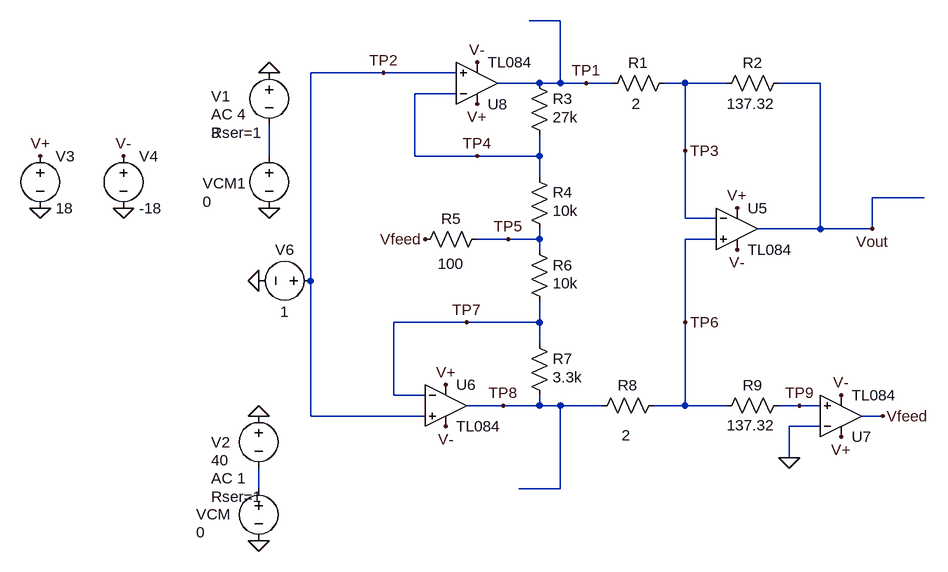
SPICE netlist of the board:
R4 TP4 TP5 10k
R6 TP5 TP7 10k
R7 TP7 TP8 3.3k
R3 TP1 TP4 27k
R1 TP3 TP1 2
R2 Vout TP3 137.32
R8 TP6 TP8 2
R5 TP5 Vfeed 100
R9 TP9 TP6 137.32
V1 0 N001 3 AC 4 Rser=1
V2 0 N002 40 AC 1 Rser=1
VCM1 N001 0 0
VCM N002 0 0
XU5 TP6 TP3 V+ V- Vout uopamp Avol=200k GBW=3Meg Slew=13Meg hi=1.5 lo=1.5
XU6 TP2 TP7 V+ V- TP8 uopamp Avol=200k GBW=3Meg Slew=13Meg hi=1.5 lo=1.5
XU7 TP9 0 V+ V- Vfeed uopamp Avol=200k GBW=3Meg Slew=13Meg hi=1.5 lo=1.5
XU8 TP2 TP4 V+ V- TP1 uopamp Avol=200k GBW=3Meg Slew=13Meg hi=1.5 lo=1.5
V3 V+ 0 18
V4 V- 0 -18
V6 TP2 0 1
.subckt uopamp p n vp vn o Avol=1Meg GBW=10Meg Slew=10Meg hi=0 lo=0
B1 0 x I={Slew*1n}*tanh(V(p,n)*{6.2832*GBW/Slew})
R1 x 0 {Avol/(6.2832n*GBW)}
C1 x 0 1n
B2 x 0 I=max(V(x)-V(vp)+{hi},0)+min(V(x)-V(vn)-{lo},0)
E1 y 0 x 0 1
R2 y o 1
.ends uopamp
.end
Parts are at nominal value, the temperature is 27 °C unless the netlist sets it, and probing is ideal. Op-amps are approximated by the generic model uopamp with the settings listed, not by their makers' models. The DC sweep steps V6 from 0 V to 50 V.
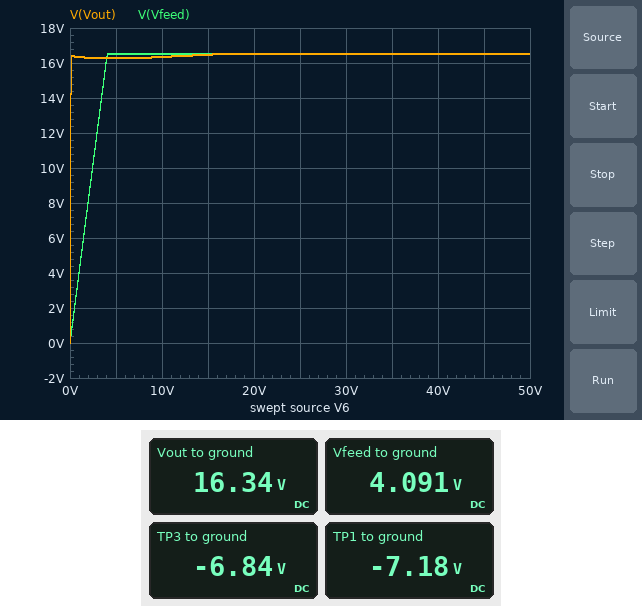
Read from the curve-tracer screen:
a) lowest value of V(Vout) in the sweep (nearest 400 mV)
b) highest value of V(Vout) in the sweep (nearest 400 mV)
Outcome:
0 V
16.4 V
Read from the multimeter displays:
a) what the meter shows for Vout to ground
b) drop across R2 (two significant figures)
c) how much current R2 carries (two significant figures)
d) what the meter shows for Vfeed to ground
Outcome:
16.34 V
23 V
170 mA
4.091 V
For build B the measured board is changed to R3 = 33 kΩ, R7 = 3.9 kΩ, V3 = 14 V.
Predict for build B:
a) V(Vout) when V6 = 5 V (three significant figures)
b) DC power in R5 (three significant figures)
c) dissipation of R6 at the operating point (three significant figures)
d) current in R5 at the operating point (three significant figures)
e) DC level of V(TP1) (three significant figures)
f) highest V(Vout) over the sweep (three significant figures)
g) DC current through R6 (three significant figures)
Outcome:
12.3 V
26.3 µW
657 µW
513 µA
-7.46 V
12.5 V
256 µA
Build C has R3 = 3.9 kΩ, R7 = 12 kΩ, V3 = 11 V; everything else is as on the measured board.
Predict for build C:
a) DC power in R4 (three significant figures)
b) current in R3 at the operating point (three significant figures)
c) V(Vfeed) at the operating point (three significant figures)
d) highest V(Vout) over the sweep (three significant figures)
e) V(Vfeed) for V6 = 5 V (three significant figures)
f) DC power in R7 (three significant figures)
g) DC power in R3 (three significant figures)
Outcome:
69.4 µW
83.3 µA
1.85 V
9.50 V
9.25 V
83.3 µW
27.1 µW
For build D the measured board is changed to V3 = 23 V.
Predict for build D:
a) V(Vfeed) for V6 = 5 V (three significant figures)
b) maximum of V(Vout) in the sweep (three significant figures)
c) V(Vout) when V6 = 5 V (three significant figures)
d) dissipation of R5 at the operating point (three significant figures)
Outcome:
20.4 V
21.5 V
21.2 V
36.7 µW
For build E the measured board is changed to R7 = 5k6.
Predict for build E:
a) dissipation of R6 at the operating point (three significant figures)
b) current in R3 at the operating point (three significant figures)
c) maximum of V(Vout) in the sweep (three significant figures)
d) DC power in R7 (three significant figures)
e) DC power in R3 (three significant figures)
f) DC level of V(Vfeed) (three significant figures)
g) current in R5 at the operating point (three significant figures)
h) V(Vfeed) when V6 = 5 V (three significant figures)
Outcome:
319 µW
179 µA
16.5 V
179 µW
861 µW
2.82 V
357 µA
14.1 V
